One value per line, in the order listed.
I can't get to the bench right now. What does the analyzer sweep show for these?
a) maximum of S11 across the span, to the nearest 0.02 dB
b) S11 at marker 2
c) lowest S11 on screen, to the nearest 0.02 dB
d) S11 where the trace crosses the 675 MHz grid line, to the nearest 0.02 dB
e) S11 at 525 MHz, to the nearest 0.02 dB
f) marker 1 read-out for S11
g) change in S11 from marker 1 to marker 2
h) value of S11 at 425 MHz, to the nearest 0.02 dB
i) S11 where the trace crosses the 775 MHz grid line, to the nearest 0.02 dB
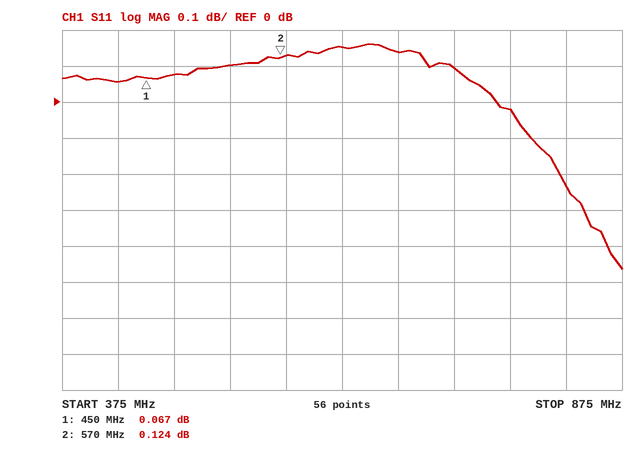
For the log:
0.16 dB
0.124 dB
-0.46 dB
0.14 dB
0.10 dB
0.067 dB
0.057 dB
0.06 dB
-0.02 dB
